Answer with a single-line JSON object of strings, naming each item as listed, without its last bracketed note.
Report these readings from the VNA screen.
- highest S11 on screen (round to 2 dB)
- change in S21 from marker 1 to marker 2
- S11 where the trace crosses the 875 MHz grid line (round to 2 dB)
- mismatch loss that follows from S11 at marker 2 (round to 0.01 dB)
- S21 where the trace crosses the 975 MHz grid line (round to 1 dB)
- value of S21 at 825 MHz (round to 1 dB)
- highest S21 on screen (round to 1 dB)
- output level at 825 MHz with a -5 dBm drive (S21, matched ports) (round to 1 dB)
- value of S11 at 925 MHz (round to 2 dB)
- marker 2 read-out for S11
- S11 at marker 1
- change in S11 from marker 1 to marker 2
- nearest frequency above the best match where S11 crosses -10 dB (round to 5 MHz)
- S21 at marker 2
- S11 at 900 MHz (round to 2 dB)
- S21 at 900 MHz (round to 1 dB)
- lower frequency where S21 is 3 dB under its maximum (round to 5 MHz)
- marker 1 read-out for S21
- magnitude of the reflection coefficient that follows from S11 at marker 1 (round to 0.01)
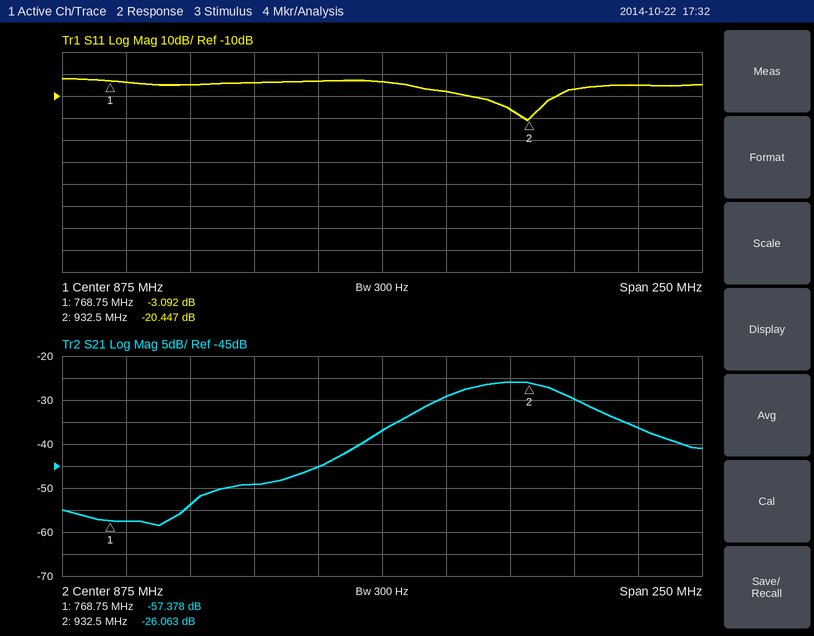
{"highest S11 on screen": "-2 dB", "change in S21 from marker 1 to marker 2": "31.315 dB", "S11 where the trace crosses the 875 MHz grid line": "-4 dB", "mismatch loss that follows from S11 at marker 2": "0.04 dB", "S21 where the trace crosses the 975 MHz grid line": "-36 dB", "value of S21 at 825 MHz": "-49 dB", "highest S21 on screen": "-26 dB", "output level at 825 MHz with a -5 dBm drive (S21, matched ports)": "-54 dBm", "value of S11 at 925 MHz": "-16 dB", "marker 2 read-out for S11": "-20.447 dB", "S11 at marker 1": "-3.092 dB", "change in S11 from marker 1 to marker 2": "-17.355 dB", "nearest frequency above the best match where S11 crosses -10 dB": "945 MHz", "S21 at marker 2": "-26.063 dB", "S11 at 900 MHz": "-8 dB", "S21 at 900 MHz": "-29 dB", "lower frequency where S21 is 3 dB under its maximum": "900 MHz", "marker 1 read-out for S21": "-57.378 dB", "magnitude of the reflection coefficient that follows from S11 at marker 1": "0.70"}
